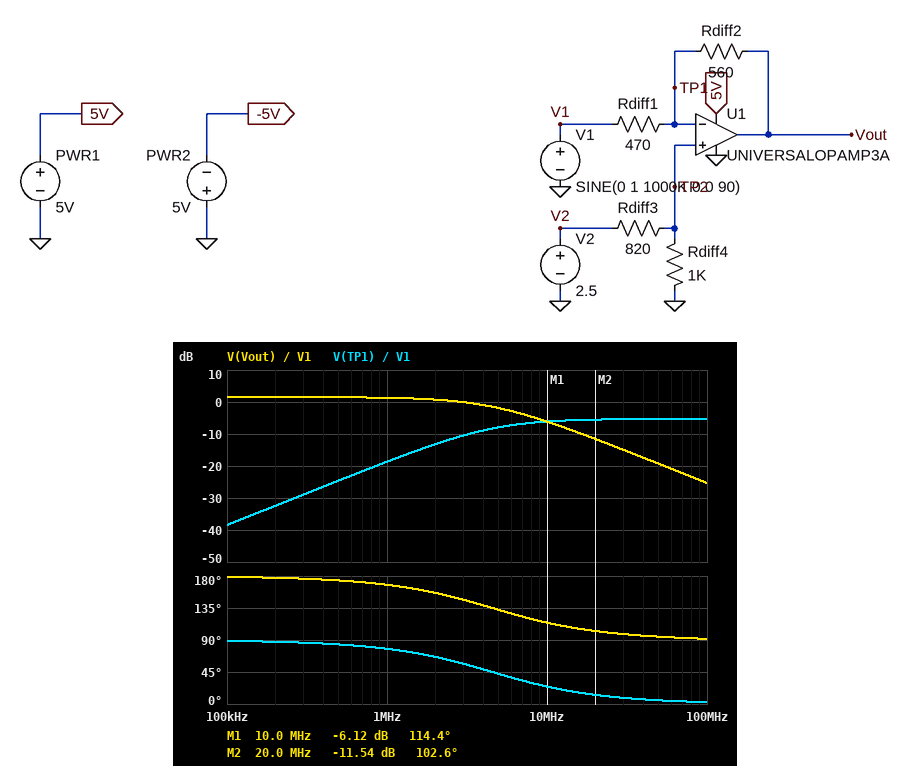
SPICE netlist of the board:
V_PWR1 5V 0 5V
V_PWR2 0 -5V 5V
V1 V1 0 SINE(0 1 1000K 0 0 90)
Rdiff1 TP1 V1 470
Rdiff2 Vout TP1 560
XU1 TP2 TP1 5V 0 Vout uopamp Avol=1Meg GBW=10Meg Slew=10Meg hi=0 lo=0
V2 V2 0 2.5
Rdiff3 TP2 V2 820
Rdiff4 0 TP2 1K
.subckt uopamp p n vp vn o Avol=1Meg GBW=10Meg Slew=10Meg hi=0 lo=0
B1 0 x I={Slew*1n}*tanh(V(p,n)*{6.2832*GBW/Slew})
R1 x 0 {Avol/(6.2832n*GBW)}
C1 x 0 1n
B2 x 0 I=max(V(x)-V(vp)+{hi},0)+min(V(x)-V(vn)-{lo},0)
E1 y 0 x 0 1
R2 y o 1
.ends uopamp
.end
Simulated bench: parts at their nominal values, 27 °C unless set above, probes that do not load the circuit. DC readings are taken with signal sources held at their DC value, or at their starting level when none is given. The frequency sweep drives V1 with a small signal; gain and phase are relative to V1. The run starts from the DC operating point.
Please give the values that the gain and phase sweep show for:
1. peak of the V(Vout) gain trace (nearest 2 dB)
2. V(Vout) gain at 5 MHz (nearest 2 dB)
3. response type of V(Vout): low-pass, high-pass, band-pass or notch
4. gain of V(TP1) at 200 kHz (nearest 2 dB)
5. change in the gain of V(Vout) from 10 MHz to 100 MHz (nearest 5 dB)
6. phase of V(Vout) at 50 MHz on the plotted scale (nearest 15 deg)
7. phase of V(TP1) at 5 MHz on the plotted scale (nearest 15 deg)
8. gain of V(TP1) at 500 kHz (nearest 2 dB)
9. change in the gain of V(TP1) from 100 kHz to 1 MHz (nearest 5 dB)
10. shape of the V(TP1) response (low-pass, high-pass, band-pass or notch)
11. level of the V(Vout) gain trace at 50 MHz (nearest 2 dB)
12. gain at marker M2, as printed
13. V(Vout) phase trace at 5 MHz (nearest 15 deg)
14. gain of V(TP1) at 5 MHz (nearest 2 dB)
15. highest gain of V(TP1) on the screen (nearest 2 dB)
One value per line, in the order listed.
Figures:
2 dB
-2 dB
low-pass
-32 dB
-20 dB
90 deg
45 deg
-24 dB
20 dB
high-pass
-20 dB
-11.54 dB
135 deg
-8 dB
-6 dB
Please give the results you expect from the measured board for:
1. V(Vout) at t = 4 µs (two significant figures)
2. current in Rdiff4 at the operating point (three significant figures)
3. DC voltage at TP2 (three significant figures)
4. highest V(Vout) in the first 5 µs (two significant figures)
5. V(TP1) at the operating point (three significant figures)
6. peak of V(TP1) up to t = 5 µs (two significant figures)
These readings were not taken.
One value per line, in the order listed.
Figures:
1.9 V
1.37 mA
1.37 V
4.2 V
1.37 V
1.5 V
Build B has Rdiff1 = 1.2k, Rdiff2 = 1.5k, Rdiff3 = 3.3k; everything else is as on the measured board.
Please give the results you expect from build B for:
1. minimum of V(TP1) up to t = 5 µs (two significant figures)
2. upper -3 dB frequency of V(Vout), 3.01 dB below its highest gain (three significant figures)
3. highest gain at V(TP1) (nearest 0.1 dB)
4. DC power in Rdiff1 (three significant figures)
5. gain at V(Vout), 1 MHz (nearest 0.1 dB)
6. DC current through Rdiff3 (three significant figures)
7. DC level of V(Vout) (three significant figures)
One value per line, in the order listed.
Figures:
430 mV
4.44 MHz
-5.1 dB
146 µW
1.7 dB
581 µA
58.1 mV
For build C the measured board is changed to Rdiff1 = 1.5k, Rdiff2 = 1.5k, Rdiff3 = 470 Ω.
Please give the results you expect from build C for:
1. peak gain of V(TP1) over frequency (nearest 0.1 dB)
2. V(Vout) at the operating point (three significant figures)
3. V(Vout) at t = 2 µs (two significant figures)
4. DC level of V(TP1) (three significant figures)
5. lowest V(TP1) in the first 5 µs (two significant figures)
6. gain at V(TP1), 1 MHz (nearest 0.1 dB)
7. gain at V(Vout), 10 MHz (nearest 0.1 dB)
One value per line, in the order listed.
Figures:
-6.0 dB
2.40 V
2.4 V
1.70 V
1.6 V
-20.2 dB
-7.0 dB
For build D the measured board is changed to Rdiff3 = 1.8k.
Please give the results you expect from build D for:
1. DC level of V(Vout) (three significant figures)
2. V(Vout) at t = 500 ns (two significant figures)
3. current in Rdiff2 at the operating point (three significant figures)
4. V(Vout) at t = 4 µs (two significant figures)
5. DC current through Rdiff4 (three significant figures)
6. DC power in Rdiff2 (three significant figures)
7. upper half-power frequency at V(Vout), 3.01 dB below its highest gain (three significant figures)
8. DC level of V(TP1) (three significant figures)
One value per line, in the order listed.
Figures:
765 mV
3.1 V
228 µA
830 mV
893 µA
29.1 µW
4.56 MHz
893 mV
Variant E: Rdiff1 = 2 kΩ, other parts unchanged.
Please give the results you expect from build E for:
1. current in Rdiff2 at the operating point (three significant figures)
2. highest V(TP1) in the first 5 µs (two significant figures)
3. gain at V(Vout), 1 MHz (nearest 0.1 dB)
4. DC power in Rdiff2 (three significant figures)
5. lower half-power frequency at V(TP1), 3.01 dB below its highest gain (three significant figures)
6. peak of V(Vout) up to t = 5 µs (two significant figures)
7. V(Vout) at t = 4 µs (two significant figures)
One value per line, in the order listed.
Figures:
187 µA
1.4 V
-11.1 dB
19.5 µW
7.81 MHz
2.0 V
1.5 V
